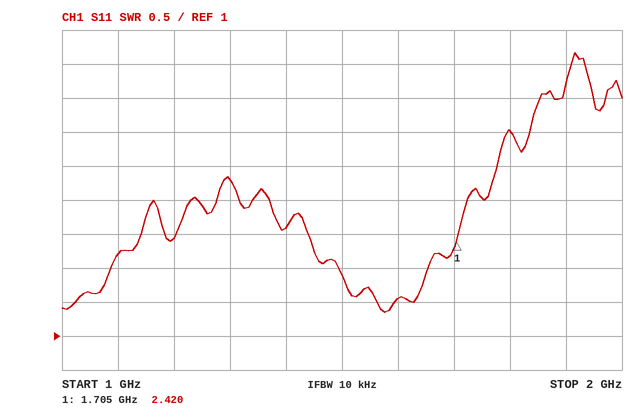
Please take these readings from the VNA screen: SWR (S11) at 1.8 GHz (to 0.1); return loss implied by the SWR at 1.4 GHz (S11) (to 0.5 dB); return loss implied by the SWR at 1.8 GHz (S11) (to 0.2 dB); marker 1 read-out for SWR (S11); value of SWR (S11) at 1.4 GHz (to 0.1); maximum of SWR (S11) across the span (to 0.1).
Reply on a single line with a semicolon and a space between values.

4.0; 7.0 dB; 4.4 dB; 2.420; 2.6; 5.2
